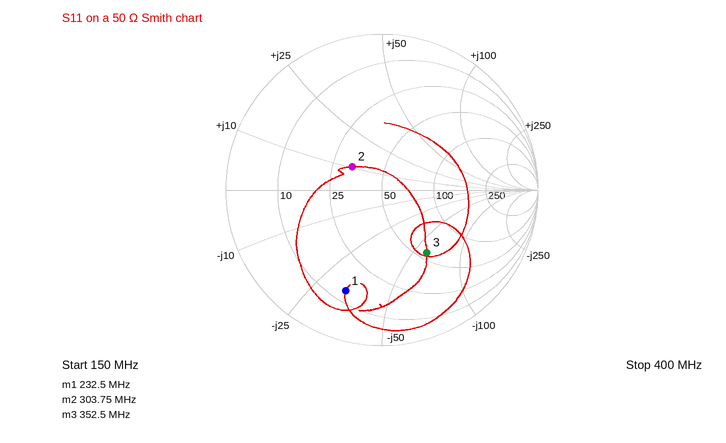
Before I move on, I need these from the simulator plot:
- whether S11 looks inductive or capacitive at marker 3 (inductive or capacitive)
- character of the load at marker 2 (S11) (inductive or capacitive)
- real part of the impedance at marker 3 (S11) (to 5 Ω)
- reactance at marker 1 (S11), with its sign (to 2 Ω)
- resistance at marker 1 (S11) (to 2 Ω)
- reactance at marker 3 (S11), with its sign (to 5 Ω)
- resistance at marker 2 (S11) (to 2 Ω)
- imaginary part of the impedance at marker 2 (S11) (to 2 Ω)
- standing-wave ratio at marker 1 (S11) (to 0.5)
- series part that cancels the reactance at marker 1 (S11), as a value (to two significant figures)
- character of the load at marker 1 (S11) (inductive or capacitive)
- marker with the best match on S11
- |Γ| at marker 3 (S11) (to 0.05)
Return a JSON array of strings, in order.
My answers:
["capacitive", "inductive", "55 Ω", "-34 Ω", "14 Ω", "-60 Ω", "32 Ω", "+10 Ω", "5.5", "23 nH", "capacitive", "marker 2", "0.50"]
